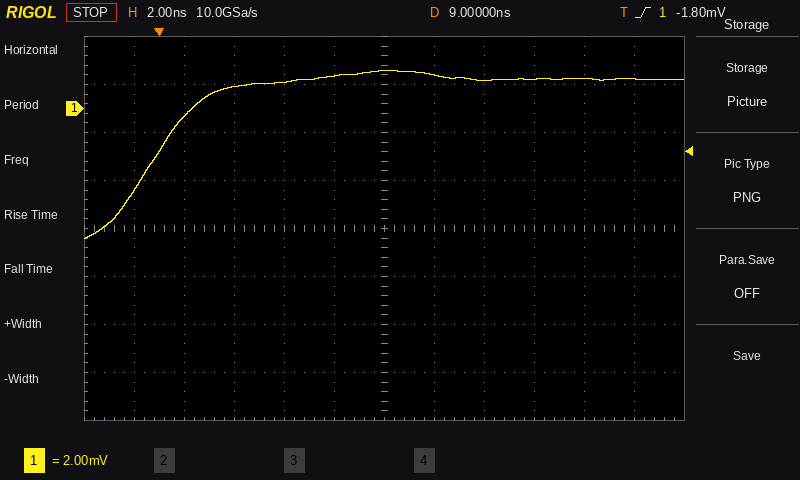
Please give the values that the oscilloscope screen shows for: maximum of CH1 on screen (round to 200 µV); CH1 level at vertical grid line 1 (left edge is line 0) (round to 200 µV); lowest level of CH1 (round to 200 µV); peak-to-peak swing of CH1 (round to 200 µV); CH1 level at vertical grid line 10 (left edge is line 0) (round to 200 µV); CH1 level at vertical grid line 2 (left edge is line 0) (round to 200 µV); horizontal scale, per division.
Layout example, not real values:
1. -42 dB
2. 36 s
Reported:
1. 1.6 mV
2. -3.4 mV
3. -5.4 mV
4. 7.0 mV
5. 1.2 mV
6. -400 µV
7. 2 ns
